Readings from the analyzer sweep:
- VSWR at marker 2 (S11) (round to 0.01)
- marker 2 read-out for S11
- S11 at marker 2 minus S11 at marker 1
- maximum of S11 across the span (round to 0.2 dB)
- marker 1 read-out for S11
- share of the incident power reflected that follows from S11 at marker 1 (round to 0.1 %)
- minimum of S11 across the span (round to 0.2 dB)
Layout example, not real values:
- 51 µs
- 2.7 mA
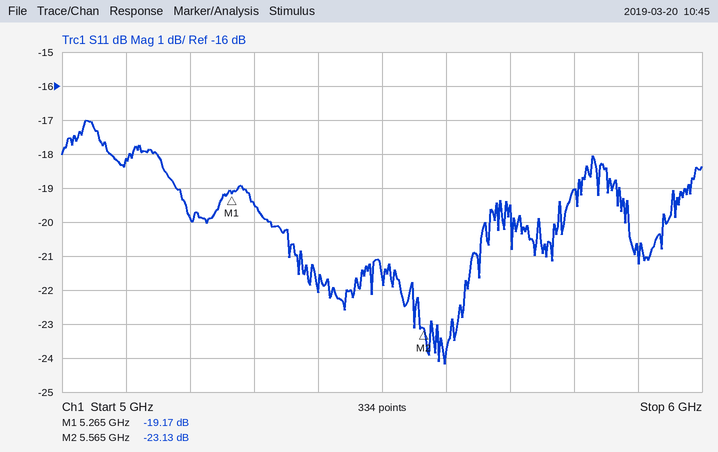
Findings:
- 1.15
- -23.13 dB
- -3.96 dB
- -17.0 dB
- -19.17 dB
- 1.2 %
- -24.2 dB
